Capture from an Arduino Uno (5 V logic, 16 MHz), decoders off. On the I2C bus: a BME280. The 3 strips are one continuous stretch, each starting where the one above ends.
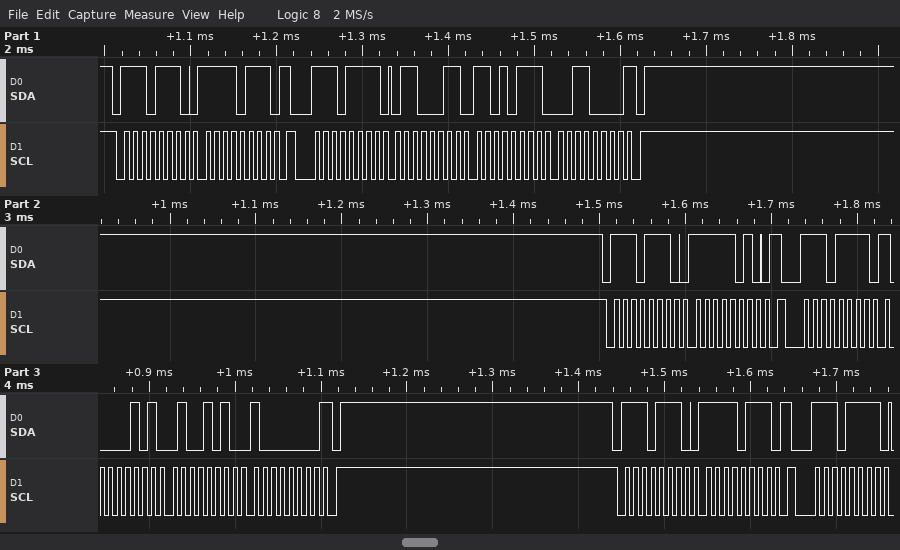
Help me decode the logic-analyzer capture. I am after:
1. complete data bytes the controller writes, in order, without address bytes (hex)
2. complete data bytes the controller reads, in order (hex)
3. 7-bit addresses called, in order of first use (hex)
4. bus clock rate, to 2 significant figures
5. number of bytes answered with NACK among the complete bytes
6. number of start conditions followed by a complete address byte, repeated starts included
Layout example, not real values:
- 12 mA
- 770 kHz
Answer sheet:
- F7 FA F7
- 63 D7 30 85 4A 80
- 0x77
- 100 kHz
- 2
- 6
